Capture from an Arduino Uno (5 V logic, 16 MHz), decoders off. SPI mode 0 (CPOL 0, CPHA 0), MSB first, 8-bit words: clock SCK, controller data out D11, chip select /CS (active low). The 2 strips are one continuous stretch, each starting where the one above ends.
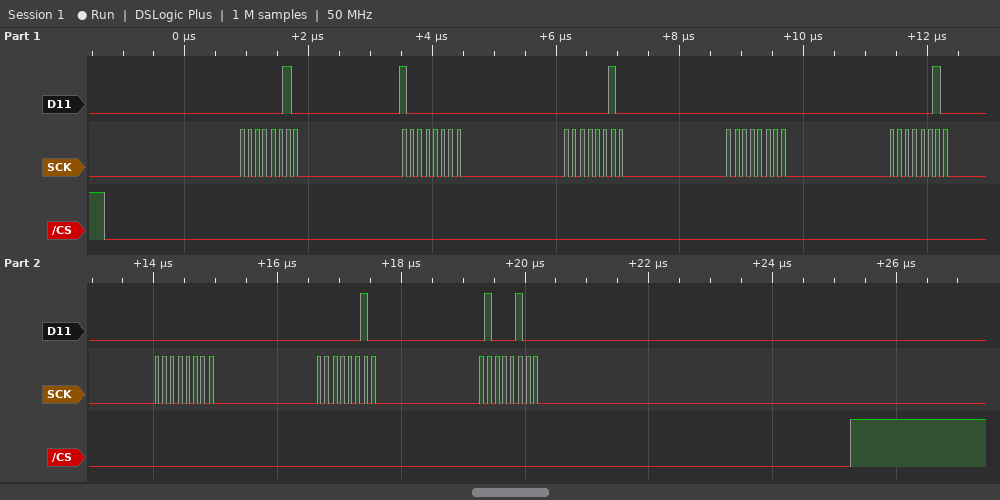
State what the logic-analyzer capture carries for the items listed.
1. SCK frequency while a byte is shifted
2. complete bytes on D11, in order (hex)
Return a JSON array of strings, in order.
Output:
["8 MHz", "0x02 0x80 0x02 0x00 0x02 0x00 0x02 0x44"]
